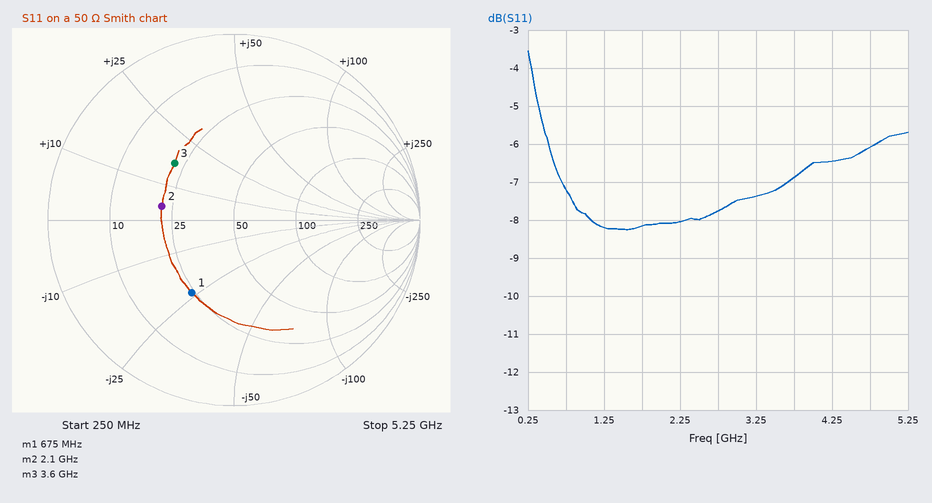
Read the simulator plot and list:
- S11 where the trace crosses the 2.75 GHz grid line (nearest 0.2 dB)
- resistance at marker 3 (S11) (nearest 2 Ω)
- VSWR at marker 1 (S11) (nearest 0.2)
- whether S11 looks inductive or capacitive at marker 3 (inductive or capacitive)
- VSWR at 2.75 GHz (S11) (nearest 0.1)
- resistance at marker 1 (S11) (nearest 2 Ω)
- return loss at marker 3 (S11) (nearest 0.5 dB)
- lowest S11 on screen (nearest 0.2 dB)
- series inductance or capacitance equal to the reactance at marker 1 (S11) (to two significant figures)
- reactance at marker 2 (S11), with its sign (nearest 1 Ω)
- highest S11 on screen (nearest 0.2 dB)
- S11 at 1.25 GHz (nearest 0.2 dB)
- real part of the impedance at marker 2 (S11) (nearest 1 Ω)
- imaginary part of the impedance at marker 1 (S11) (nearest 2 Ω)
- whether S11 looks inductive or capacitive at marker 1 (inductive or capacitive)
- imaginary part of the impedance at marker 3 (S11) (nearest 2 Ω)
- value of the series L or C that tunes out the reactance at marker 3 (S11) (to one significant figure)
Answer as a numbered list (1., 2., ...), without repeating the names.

1. -7.8 dB
2. 22 Ω
3. 2.6
4. inductive
5. 2.4
6. 24 Ω
7. 7.0 dB
8. -8.2 dB
9. 10 pF
10. +4 Ω
11. -3.6 dB
12. -8.2 dB
13. 22 Ω
14. -24 Ω
15. capacitive
16. +16 Ω
17. 3 pF
